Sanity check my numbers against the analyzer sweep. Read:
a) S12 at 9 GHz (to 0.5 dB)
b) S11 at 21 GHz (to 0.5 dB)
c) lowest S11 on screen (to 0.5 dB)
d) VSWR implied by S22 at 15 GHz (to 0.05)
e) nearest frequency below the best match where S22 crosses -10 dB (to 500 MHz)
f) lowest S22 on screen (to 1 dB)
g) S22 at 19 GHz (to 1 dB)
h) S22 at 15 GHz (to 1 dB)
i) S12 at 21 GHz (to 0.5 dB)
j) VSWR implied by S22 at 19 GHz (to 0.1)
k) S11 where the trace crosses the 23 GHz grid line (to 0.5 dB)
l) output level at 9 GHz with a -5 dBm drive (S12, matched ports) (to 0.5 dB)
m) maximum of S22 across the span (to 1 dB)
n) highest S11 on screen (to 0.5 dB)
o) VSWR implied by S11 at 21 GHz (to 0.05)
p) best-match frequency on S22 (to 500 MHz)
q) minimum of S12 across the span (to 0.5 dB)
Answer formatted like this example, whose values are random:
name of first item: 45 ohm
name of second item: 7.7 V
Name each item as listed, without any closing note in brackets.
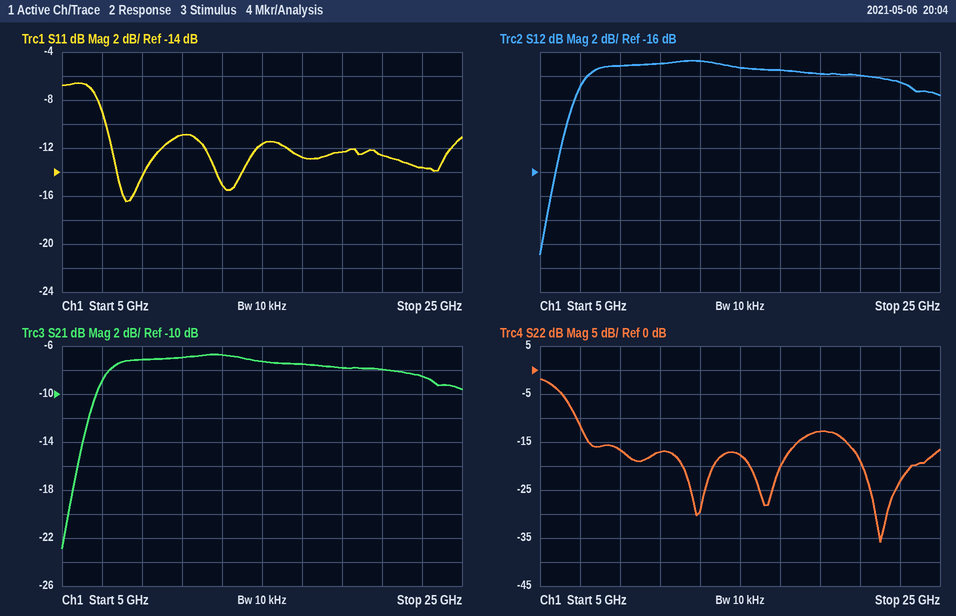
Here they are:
S12 at 9 GHz: -7.0 dB
S11 at 21 GHz: -12.5 dB
lowest S11 on screen: -16.5 dB
VSWR implied by S22 at 15 GHz: 1.30
nearest frequency below the best match where S22 crosses -10 dB: 7.0 GHz
lowest S22 on screen: -36 dB
S22 at 19 GHz: -13 dB
S22 at 15 GHz: -18 dB
S12 at 21 GHz: -8.0 dB
VSWR implied by S22 at 19 GHz: 1.6
S11 where the trace crosses the 23 GHz grid line: -13.5 dB
output level at 9 GHz with a -5 dBm drive (S12, matched ports): -12.0 dBm
maximum of S22 across the span: -2 dB
highest S11 on screen: -6.5 dB
VSWR implied by S11 at 21 GHz: 1.60
best-match frequency on S22: 22.0 GHz
minimum of S12 across the span: -23.0 dB
